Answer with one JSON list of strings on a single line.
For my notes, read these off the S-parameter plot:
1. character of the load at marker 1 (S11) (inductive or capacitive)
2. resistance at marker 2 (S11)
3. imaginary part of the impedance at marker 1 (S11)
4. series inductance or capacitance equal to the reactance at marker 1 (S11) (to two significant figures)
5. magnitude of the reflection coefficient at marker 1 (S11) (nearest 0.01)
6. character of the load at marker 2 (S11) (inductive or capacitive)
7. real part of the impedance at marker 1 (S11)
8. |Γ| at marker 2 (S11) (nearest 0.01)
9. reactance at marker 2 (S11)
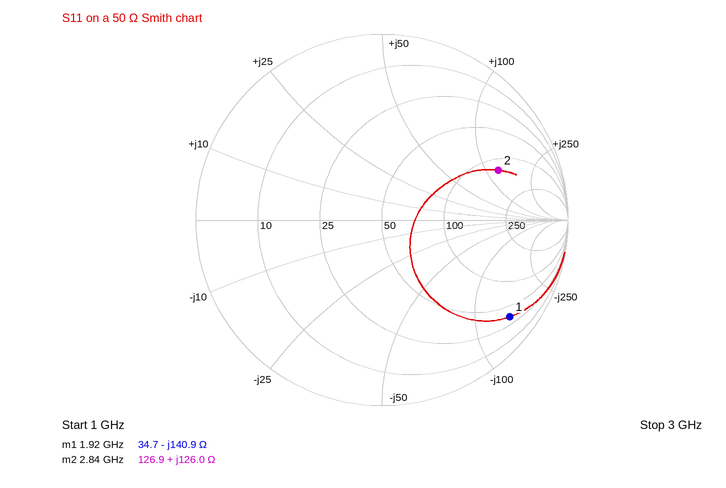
["capacitive", "126.9 Ω", "-140.9 Ω", "590 fF", "0.86", "inductive", "34.7 Ω", "0.68", "+126.0 Ω"]
